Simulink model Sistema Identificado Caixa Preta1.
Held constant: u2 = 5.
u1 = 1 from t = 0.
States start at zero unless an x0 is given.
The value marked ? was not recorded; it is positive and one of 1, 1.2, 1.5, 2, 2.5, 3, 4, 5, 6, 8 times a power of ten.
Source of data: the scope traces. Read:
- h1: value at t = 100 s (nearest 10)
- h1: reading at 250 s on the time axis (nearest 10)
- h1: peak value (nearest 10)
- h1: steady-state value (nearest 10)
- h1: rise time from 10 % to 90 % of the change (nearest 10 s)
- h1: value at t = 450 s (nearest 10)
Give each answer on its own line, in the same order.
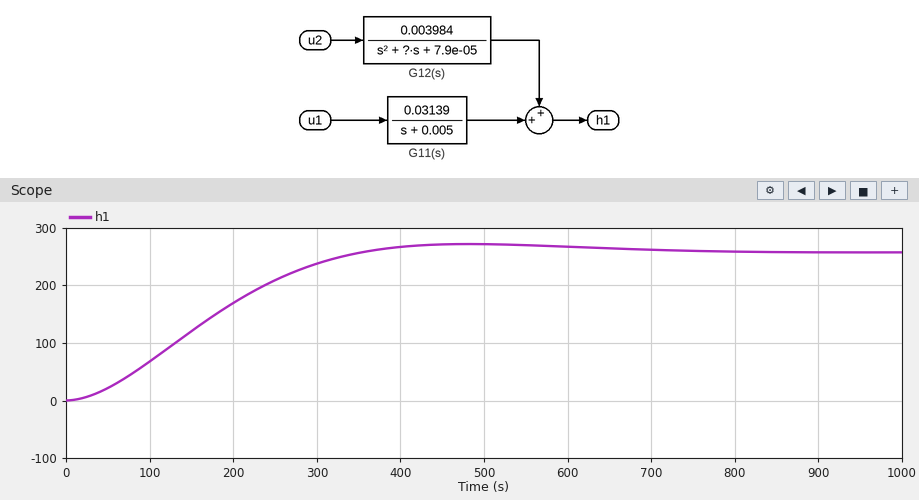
70
210
270
260
230 s
270
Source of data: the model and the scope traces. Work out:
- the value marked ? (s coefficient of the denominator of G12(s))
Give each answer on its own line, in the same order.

0.012
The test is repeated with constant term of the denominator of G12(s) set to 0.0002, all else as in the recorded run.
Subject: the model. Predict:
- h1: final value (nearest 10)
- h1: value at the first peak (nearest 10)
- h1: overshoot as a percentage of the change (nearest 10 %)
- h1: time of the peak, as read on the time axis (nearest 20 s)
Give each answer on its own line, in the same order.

110
130
20 %
240 s
